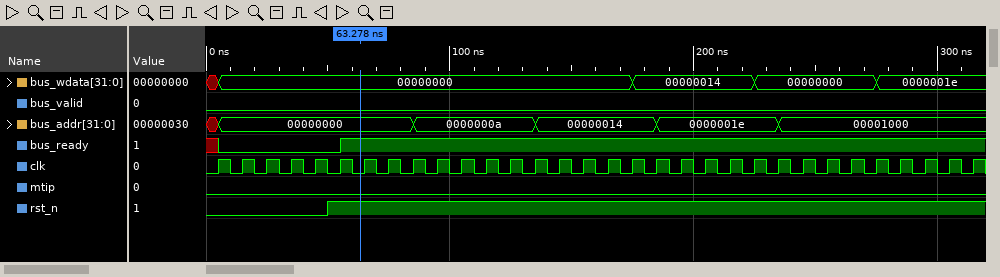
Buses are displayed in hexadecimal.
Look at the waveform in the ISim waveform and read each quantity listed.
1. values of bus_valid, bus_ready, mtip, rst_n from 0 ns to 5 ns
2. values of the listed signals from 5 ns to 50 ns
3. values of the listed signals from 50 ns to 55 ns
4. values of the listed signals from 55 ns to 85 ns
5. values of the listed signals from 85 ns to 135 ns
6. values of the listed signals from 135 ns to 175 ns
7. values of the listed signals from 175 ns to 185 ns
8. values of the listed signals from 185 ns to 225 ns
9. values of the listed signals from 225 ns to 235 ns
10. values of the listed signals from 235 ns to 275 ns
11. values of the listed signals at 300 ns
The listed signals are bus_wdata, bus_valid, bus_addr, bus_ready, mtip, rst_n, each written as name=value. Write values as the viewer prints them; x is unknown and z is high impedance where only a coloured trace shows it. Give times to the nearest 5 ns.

bus_valid=0, bus_ready=x, mtip=0, rst_n=0
bus_wdata=00000000, bus_valid=0, bus_addr=00000000, bus_ready=0, mtip=0, rst_n=0
bus_wdata=00000000, bus_valid=0, bus_addr=00000000, bus_ready=0, mtip=0, rst_n=1
bus_wdata=00000000, bus_valid=0, bus_addr=00000000, bus_ready=1, mtip=0, rst_n=1
bus_wdata=00000000, bus_valid=0, bus_addr=0000000a, bus_ready=1, mtip=0, rst_n=1
bus_wdata=00000000, bus_valid=0, bus_addr=00000014, bus_ready=1, mtip=0, rst_n=1
bus_wdata=00000014, bus_valid=0, bus_addr=00000014, bus_ready=1, mtip=0, rst_n=1
bus_wdata=00000014, bus_valid=0, bus_addr=0000001e, bus_ready=1, mtip=0, rst_n=1
bus_wdata=00000000, bus_valid=0, bus_addr=0000001e, bus_ready=1, mtip=0, rst_n=1
bus_wdata=00000000, bus_valid=0, bus_addr=00001000, bus_ready=1, mtip=0, rst_n=1
bus_wdata=0000001e, bus_valid=0, bus_addr=00001000, bus_ready=1, mtip=0, rst_n=1
